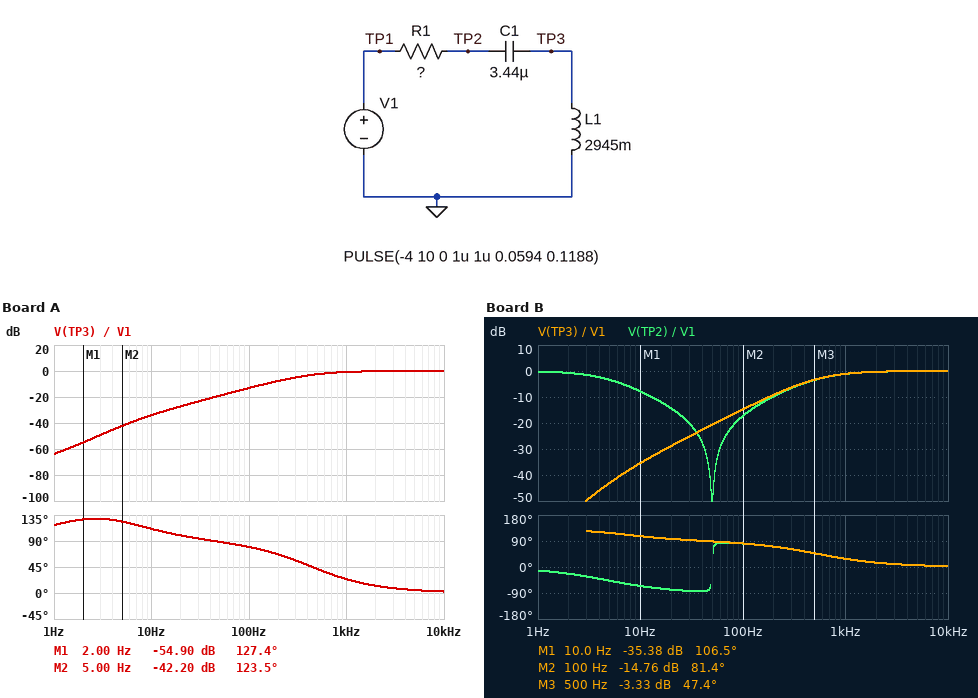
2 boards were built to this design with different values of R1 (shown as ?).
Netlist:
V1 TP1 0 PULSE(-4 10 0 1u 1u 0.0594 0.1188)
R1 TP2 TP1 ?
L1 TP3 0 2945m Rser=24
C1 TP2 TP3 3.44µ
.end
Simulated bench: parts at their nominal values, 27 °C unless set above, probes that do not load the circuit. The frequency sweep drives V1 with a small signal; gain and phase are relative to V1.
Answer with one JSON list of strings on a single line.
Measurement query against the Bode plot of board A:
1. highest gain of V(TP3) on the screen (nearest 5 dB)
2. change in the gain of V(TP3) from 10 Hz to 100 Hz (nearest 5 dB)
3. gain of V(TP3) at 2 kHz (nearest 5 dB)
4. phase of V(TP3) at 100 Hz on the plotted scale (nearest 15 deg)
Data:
["0 dB", "20 dB", "0 dB", "75 deg"]
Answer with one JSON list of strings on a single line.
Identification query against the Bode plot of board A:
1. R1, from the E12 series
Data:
["8.2 kΩ"]
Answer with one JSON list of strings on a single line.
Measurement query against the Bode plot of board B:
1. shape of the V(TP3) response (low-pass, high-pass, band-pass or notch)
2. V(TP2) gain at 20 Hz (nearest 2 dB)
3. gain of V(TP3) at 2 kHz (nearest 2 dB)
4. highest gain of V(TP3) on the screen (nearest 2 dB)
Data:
["high-pass", "-14 dB", "0 dB", "0 dB"]
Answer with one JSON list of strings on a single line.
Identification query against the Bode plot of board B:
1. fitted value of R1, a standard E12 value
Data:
["10 kΩ"]
